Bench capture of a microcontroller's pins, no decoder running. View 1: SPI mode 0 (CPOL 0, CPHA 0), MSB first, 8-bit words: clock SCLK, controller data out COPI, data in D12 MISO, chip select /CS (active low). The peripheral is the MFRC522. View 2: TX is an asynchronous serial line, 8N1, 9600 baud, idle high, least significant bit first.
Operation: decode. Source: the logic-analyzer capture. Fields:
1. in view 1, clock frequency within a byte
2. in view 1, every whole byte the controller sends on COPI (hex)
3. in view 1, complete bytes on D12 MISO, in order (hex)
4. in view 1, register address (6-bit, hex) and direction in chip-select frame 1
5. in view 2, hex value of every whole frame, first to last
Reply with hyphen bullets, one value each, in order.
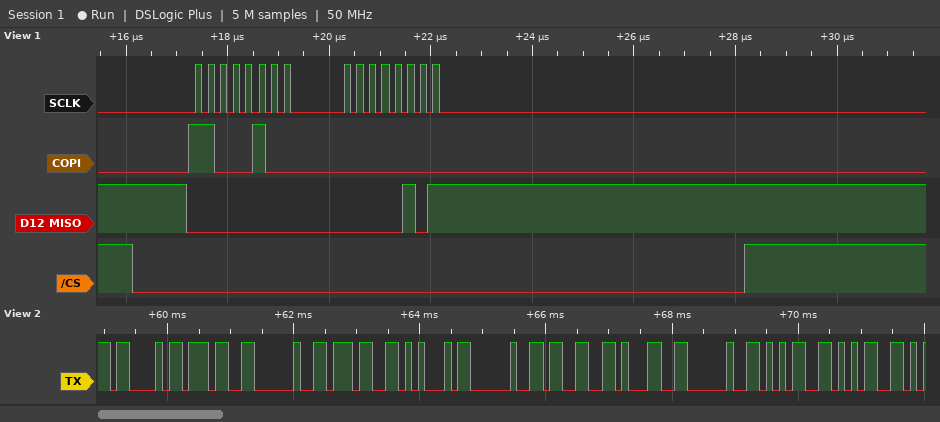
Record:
- 4 MHz
- 0xC4 0x00
- 0x00 0x05
- 0x22 read
- 43 37 20 37 45 20 33 31 20 35 35
